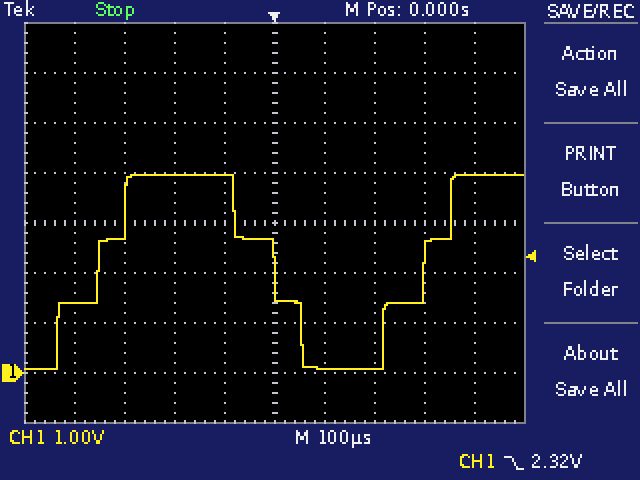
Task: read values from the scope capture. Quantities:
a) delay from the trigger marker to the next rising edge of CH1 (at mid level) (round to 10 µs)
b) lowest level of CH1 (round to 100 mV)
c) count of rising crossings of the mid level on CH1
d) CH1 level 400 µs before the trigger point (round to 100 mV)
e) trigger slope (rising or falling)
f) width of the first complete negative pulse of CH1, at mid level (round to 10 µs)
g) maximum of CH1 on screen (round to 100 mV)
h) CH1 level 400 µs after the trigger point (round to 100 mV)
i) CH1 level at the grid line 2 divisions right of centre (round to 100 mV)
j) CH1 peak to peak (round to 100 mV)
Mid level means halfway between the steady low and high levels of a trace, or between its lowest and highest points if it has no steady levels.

300 µs
100 mV
2
1.4 V
falling
300 µs
4.0 V
4.0 V
100 mV
3.9 V
